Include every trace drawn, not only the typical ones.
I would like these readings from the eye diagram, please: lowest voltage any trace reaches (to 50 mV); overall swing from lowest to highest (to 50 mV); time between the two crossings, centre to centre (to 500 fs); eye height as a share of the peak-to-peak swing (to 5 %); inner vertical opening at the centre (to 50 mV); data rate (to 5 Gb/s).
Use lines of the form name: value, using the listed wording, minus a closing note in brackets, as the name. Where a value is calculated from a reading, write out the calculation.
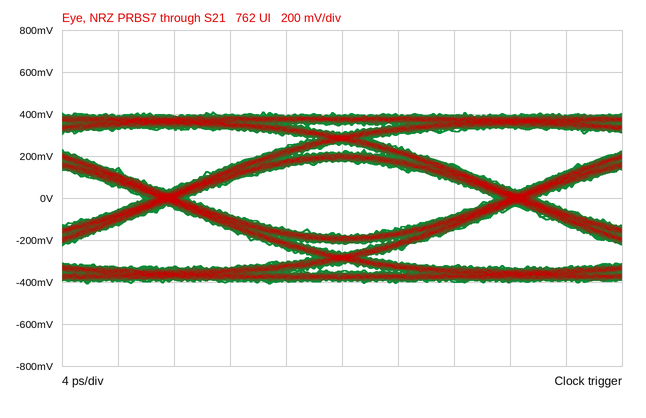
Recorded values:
lowest voltage any trace reaches: -400 mV
overall swing from lowest to highest: 800 mV
time between the two crossings, centre to centre: 25.0 ps
eye height as a share of the peak-to-peak swing: 350 mV / 800 mV ≈ 43.8 %, so 45 % to the nearest 5 %
inner vertical opening at the centre: 350 mV
data rate: 40 Gb/s
